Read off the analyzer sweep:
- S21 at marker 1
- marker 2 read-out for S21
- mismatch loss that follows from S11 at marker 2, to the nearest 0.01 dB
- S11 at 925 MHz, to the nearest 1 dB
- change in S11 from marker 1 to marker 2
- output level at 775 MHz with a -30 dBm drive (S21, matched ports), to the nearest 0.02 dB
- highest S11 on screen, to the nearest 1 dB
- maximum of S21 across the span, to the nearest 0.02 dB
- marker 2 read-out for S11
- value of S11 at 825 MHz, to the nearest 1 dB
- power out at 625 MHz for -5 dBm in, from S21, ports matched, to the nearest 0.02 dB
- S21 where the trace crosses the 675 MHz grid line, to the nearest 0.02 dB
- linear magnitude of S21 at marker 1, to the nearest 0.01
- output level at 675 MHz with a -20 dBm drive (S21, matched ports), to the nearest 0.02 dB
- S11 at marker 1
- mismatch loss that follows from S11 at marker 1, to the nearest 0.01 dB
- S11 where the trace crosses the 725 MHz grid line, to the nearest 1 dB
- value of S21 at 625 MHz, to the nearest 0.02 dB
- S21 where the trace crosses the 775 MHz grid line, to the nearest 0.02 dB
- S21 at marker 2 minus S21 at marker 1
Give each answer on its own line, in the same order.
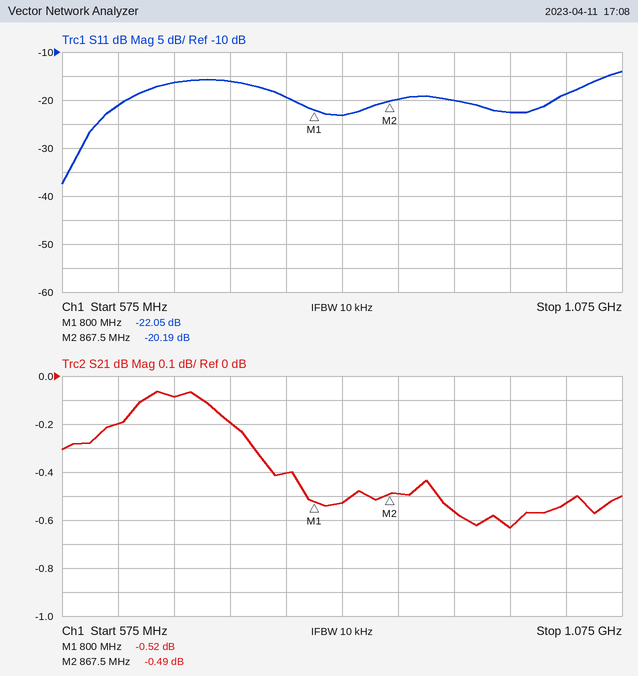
-0.52 dB
-0.49 dB
0.04 dB
-20 dB
1.86 dB
-30.40 dBm
-14 dB
-0.06 dB
-20.19 dB
-23 dB
-5.20 dBm
-0.08 dB
0.94
-20.08 dBm
-22.05 dB
0.03 dB
-16 dB
-0.20 dB
-0.40 dB
0.03 dB
